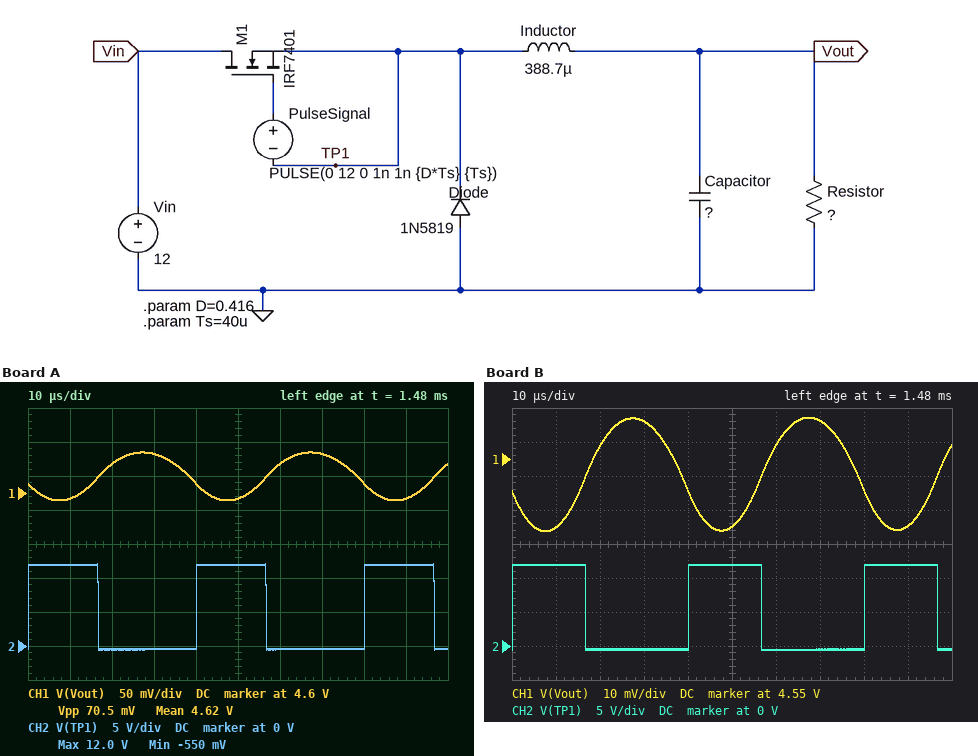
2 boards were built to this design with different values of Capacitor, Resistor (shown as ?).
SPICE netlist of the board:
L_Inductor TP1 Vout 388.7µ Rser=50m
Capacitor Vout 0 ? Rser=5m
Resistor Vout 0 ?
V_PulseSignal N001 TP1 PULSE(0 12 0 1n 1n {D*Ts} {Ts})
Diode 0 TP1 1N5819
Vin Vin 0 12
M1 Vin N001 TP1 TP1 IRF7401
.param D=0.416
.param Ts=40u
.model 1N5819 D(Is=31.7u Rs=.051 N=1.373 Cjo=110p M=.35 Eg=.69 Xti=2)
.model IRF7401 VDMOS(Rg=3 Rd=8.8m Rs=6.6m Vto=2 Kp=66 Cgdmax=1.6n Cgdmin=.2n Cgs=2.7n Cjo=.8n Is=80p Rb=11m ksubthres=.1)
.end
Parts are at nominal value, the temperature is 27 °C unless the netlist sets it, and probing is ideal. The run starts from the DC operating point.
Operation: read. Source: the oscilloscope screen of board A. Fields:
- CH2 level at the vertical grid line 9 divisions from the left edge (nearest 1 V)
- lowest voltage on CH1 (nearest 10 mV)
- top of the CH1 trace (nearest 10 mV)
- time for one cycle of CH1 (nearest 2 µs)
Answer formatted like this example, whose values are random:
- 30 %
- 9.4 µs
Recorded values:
- 12 V
- 4.59 V
- 4.66 V
- 40 µs
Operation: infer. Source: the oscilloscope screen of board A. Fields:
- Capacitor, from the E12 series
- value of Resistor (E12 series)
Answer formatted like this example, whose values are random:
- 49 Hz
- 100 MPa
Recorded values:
- 22 µF
- 2.7 Ω
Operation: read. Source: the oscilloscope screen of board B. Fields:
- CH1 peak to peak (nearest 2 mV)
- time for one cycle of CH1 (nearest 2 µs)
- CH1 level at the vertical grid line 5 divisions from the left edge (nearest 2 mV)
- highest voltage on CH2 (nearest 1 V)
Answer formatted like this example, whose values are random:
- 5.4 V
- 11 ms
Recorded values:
- 34 mV
- 40 µs
- 4.530 V
- 12 V
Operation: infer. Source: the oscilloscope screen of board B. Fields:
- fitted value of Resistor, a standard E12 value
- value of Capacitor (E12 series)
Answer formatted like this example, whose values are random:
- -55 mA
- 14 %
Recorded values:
- 1.8 Ω
- 47 µF
